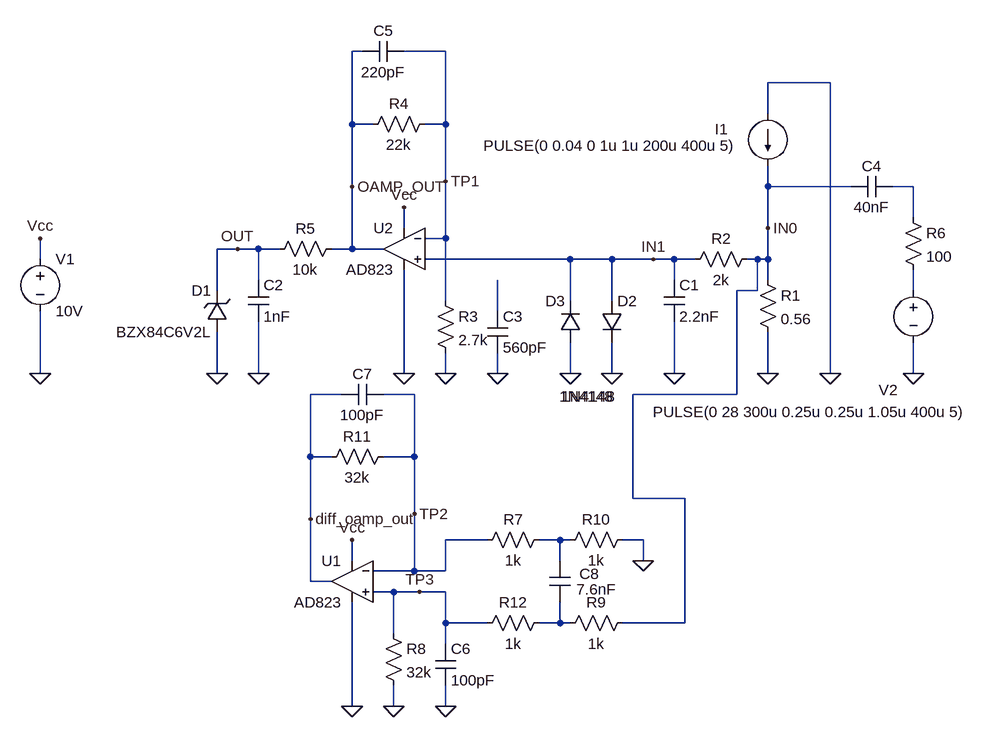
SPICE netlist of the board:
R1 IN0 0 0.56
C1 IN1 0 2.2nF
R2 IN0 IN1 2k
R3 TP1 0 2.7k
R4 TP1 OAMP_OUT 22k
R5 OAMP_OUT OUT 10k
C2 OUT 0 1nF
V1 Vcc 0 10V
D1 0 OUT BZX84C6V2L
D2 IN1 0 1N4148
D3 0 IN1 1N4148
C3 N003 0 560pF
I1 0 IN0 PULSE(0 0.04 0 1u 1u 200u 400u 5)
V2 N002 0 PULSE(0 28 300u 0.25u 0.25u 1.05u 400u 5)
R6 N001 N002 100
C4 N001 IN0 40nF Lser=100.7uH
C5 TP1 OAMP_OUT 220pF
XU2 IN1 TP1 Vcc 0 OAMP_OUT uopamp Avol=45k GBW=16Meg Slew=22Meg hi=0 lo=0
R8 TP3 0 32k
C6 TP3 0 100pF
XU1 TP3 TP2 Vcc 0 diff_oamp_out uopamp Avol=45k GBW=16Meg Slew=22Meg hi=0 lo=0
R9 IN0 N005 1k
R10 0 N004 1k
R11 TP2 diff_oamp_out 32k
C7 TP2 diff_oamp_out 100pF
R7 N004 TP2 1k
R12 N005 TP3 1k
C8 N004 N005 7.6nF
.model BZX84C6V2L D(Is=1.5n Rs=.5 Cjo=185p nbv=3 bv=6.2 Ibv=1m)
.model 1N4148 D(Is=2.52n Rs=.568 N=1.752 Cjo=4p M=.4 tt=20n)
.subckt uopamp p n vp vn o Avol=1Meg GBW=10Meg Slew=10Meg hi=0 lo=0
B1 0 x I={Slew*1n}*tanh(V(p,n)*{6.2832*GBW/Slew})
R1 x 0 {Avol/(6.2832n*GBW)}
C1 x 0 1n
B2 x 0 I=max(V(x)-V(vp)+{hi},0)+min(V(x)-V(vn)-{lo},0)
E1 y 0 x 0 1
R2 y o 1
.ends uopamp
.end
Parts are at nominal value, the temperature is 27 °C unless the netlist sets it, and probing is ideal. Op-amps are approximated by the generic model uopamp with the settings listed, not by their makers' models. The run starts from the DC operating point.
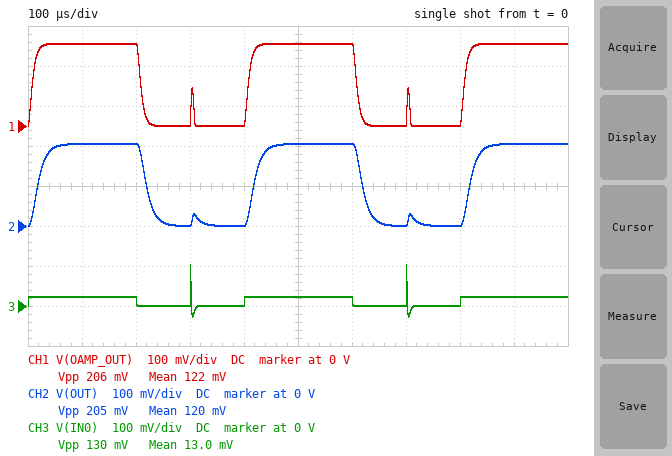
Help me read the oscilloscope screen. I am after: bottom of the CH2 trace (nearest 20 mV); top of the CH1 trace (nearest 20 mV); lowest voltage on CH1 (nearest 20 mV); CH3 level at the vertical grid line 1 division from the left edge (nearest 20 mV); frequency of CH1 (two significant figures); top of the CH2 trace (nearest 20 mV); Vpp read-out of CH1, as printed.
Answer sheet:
0 V
200 mV
0 V
20 mV
2.5 kHz
200 mV
206 mV
